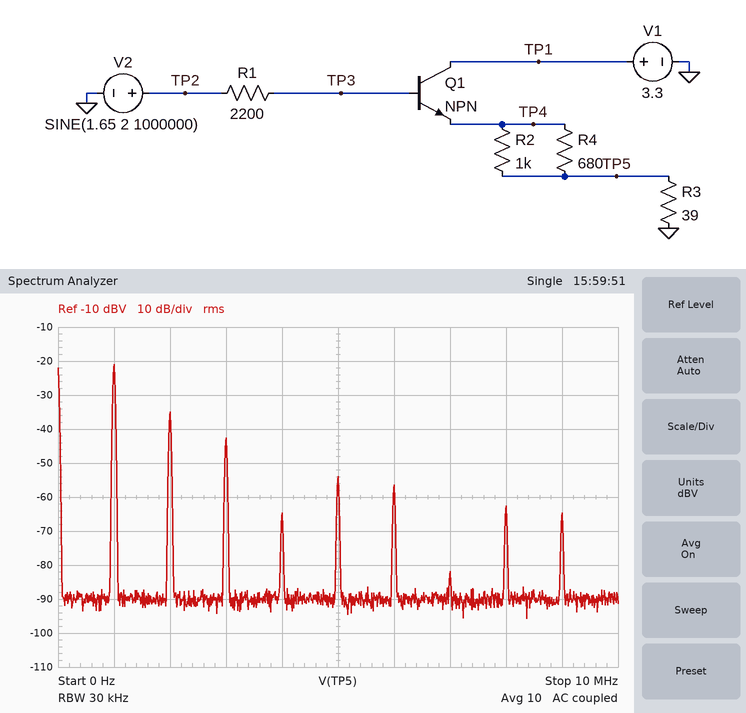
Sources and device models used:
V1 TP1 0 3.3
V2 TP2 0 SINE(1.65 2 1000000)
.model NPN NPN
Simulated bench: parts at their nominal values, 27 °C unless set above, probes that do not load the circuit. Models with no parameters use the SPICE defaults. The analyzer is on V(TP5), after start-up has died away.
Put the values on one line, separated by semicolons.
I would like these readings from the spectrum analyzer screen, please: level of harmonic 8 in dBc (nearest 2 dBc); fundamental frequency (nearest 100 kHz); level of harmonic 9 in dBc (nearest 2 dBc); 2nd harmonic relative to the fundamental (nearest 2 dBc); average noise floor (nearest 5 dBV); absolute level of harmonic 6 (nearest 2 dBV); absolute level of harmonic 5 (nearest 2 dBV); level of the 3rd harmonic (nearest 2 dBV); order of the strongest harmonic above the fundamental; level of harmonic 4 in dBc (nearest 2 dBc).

-42 dBc; 1.0 MHz; -44 dBc; -14 dBc; -90 dBV; -56 dBV; -54 dBV; -42 dBV; 2; -44 dBc
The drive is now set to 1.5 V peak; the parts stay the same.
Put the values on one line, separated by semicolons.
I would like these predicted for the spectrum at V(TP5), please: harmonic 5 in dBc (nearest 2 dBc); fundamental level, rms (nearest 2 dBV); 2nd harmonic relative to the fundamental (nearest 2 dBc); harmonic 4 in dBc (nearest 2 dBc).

-56 dBc; -22 dBV; -18 dBc; -32 dBc
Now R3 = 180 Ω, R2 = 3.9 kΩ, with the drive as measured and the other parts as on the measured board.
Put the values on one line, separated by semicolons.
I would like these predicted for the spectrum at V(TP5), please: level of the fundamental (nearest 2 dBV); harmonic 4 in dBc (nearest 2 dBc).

-12 dBV; -42 dBc
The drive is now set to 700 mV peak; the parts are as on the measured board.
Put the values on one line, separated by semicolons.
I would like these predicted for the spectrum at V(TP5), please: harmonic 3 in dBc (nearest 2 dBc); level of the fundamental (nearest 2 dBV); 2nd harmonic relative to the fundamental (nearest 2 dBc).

-52 dBc; -28 dBV; -42 dBc
